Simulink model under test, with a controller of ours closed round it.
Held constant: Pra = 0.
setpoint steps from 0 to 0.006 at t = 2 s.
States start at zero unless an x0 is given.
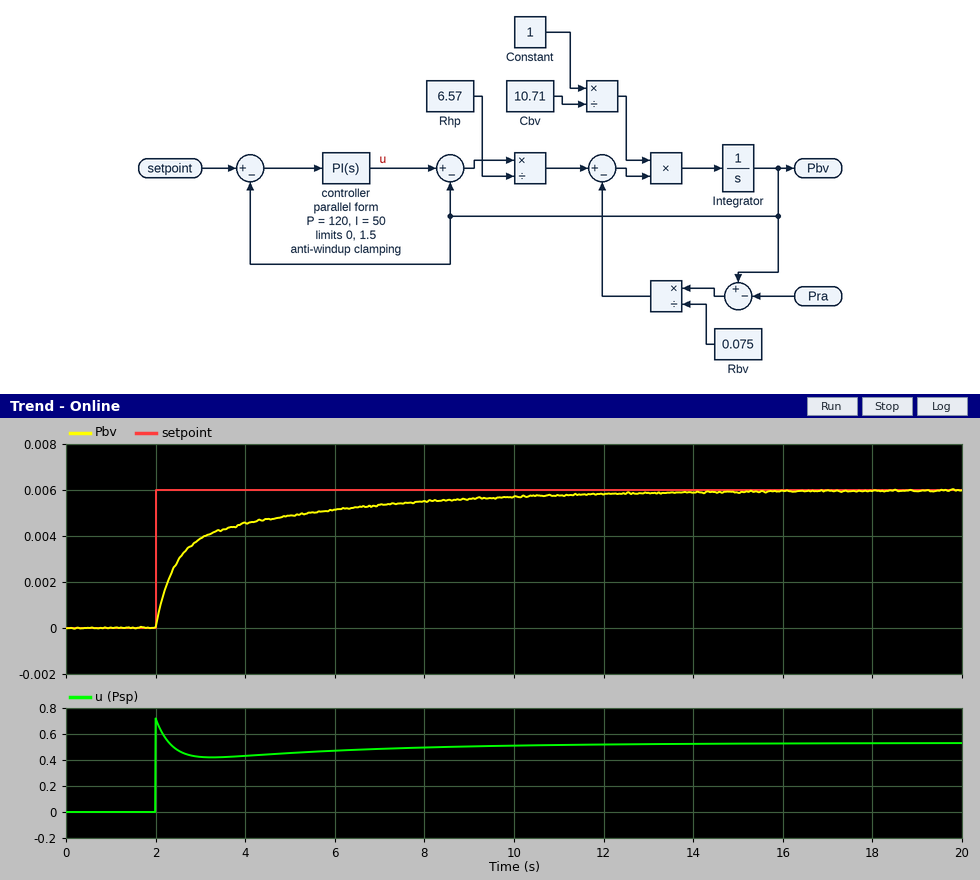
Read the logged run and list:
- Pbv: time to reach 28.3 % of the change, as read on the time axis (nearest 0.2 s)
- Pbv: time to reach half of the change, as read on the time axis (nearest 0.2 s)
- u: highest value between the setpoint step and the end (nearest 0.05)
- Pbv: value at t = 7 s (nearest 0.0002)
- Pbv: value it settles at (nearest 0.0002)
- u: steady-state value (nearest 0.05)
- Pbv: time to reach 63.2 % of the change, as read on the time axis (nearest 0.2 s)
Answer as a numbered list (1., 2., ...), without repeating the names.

1. 2.2 s
2. 2.6 s
3. 0.70
4. 0.0054
5. 0.0060
6. 0.55
7. 3.0 s
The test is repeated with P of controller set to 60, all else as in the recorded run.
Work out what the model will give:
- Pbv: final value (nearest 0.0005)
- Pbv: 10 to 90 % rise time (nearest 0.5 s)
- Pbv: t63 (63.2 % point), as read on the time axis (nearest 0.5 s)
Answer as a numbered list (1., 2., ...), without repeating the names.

1. 0.0060
2. 4.5 s
3. 3.5 s
